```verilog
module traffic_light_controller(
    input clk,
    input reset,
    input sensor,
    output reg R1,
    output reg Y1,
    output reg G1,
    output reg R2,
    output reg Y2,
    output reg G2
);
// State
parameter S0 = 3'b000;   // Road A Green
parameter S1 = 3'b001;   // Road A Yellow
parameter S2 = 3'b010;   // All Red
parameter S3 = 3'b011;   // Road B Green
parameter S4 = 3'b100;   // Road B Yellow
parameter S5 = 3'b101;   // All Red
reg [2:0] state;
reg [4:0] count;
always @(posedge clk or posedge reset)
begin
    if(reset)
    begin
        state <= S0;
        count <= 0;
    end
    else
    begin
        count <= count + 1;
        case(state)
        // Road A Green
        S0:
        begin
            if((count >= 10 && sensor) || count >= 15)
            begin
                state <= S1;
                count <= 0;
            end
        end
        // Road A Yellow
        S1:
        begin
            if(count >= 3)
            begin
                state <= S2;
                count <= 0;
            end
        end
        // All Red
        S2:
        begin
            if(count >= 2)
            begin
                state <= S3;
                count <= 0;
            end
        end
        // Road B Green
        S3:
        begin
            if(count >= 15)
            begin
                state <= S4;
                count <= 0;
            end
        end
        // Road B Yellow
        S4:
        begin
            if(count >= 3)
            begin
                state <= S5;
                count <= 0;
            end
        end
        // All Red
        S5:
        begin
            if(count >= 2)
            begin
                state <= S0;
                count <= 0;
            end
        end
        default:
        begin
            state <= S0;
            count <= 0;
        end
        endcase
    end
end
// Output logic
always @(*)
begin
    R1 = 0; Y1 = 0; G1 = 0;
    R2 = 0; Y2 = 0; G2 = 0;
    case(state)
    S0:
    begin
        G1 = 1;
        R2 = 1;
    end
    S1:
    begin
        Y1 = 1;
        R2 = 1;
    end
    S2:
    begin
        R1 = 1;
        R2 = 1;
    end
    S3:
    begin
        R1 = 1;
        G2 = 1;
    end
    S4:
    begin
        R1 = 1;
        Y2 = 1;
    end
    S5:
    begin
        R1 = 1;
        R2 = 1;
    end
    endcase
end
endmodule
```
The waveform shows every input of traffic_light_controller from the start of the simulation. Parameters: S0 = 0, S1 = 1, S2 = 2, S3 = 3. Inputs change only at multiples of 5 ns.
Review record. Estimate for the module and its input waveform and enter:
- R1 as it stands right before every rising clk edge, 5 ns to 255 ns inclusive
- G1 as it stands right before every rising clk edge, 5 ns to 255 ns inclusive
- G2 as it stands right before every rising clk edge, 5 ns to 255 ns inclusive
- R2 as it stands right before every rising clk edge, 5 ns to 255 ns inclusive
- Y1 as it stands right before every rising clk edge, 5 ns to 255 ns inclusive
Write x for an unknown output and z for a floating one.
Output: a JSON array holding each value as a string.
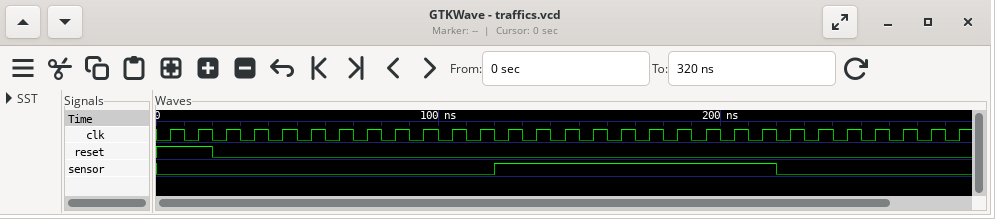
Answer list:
["0 0 0 0 0 0 0 0 0 0 0 0 0 0 0 0 0 1 1 1 1 1 1 1 1 1", "1 1 1 1 1 1 1 1 1 1 1 1 1 0 0 0 0 0 0 0 0 0 0 0 0 0", "0 0 0 0 0 0 0 0 0 0 0 0 0 0 0 0 0 0 0 0 1 1 1 1 1 1", "1 1 1 1 1 1 1 1 1 1 1 1 1 1 1 1 1 1 1 1 0 0 0 0 0 0", "0 0 0 0 0 0 0 0 0 0 0 0 0 1 1 1 1 0 0 0 0 0 0 0 0 0"]
